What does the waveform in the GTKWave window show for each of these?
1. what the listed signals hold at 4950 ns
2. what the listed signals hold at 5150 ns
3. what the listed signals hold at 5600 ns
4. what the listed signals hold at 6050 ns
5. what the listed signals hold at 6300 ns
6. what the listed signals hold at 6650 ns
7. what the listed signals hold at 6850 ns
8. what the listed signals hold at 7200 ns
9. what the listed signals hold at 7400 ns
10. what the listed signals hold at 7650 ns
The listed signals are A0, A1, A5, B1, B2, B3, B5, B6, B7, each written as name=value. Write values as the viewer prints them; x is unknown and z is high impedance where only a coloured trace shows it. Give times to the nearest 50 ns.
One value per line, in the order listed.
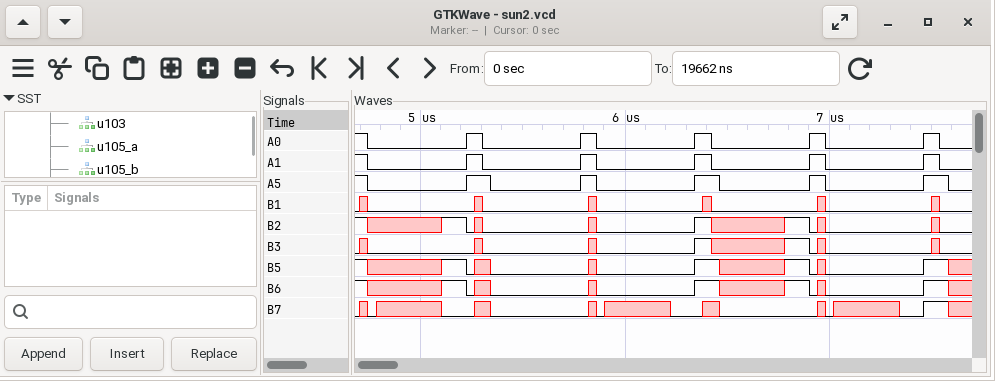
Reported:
A0=0, A1=0, A5=0, B1=0, B2=x, B3=0, B5=x, B6=x, B7=x
A0=0, A1=0, A5=0, B1=0, B2=1, B3=0, B5=1, B6=1, B7=0
A0=0, A1=0, A5=0, B1=0, B2=0, B3=0, B5=0, B6=0, B7=0
A0=0, A1=0, A5=0, B1=0, B2=0, B3=0, B5=0, B6=0, B7=x
A0=0, A1=0, A5=0, B1=0, B2=0, B3=0, B5=0, B6=0, B7=0
A0=0, A1=0, A5=0, B1=0, B2=x, B3=x, B5=x, B6=x, B7=0
A0=0, A1=0, A5=0, B1=0, B2=1, B3=1, B5=1, B6=1, B7=0
A0=0, A1=0, A5=0, B1=0, B2=0, B3=0, B5=0, B6=0, B7=x
A0=0, A1=0, A5=0, B1=0, B2=0, B3=0, B5=0, B6=0, B7=0
A0=0, A1=0, A5=0, B1=0, B2=0, B3=0, B5=x, B6=x, B7=x
